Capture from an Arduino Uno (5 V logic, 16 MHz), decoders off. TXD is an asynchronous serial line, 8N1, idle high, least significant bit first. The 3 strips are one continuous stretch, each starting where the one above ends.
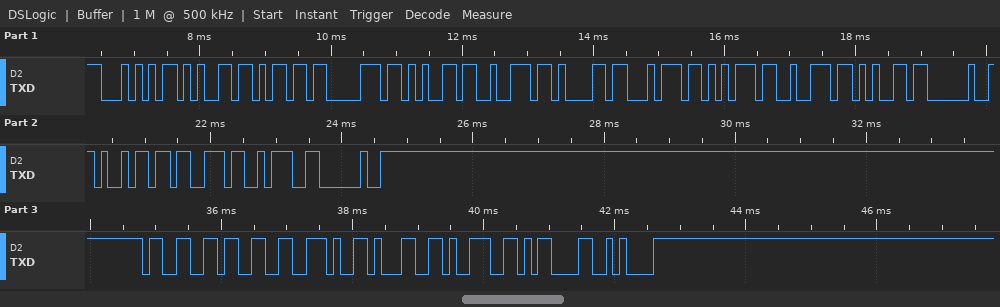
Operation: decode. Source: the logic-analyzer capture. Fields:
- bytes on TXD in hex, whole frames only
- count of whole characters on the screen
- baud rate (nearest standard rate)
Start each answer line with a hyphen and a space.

- 54 65 6D 70 65 72 61 74 75 72 65 20 69 73 3A 20 33 33 2E 31 39 0D 0A
- 23
- 9600 baud
